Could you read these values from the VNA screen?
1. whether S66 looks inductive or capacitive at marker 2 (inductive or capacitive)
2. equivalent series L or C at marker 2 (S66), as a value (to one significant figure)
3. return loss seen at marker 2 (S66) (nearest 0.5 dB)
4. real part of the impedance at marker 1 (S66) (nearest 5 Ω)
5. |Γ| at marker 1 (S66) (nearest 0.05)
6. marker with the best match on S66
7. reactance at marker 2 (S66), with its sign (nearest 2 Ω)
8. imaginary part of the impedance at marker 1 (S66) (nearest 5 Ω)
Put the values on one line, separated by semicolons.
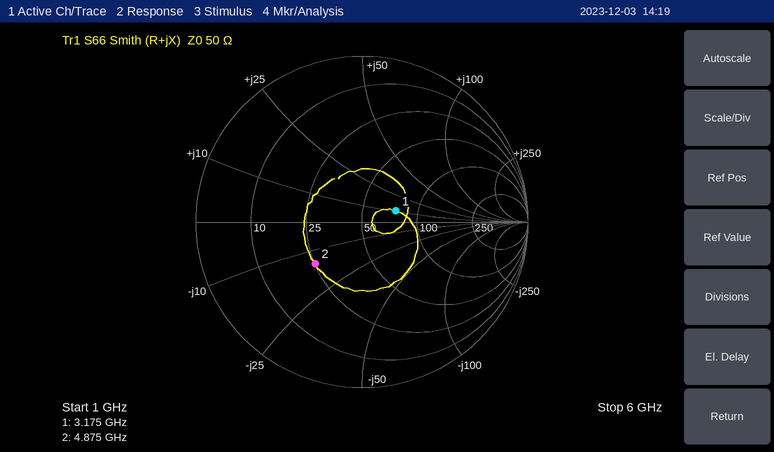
capacitive; 2 pF; 8.5 dB; 75 Ω; 0.20; marker 1; -14 Ω; +10 Ω
